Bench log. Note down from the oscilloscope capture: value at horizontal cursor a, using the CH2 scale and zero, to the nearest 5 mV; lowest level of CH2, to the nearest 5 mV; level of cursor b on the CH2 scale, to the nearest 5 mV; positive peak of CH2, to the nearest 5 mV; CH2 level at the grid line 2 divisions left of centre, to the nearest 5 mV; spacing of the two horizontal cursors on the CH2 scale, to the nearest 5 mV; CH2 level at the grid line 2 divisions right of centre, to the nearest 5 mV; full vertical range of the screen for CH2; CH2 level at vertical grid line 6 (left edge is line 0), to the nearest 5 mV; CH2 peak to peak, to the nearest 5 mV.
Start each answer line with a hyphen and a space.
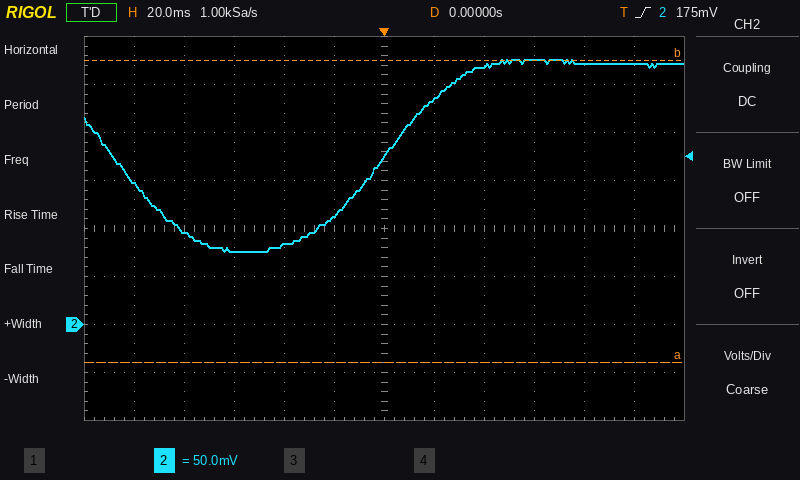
- -40 mV
- 75 mV
- 275 mV
- 275 mV
- 85 mV
- 315 mV
- 270 mV
- 400 mV
- 175 mV
- 200 mV
